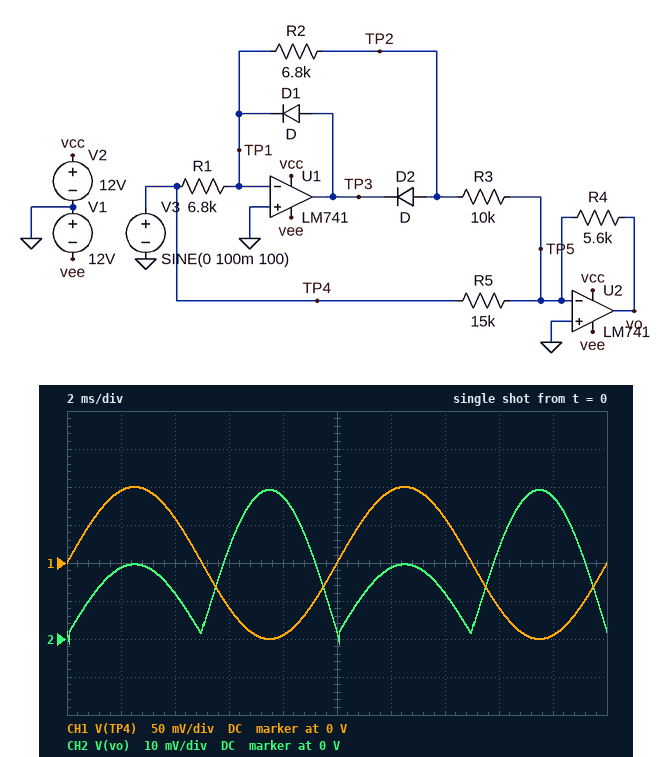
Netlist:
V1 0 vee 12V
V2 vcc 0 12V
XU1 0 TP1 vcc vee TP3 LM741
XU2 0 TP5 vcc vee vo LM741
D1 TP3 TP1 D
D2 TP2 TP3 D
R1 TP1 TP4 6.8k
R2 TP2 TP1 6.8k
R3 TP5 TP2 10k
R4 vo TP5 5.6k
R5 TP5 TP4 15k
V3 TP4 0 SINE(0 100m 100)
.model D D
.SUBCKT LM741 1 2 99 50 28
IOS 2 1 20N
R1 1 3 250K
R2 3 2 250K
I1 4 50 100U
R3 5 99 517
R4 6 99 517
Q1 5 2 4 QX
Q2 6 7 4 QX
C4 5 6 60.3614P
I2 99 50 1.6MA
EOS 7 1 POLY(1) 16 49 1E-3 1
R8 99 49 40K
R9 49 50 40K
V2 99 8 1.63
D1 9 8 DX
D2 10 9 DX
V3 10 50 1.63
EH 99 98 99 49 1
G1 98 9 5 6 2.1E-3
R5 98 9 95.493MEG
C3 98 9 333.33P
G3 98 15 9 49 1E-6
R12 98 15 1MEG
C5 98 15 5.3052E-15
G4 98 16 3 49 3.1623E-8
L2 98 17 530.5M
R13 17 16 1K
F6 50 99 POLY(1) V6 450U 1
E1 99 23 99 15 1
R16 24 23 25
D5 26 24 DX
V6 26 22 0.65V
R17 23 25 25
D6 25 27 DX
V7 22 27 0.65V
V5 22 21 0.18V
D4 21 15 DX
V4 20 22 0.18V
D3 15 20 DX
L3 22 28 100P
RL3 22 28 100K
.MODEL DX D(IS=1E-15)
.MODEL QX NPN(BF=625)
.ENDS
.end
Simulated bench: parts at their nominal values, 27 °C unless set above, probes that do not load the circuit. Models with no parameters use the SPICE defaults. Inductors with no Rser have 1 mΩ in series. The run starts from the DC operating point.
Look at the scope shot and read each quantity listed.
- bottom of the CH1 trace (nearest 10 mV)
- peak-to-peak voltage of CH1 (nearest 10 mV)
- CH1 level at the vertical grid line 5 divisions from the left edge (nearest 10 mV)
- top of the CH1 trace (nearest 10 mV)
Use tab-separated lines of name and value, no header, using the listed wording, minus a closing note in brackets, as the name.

bottom of the CH1 trace	-100 mV
peak-to-peak voltage of CH1	200 mV
CH1 level at the vertical grid line 5 divisions from the left edge	0 V
top of the CH1 trace	100 mV
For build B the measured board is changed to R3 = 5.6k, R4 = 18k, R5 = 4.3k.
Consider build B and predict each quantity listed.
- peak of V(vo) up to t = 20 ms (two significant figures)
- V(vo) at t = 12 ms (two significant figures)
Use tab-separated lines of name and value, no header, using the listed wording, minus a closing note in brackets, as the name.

peak of V(vo) up to t = 20 ms	430 mV
V(vo) at t = 12 ms	-91 mV
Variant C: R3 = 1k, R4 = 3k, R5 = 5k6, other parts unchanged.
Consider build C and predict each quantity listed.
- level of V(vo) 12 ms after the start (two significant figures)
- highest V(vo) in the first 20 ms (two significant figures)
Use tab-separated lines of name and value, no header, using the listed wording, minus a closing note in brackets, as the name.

level of V(vo) 12 ms after the start	230 mV
highest V(vo) in the first 20 ms	240 mV
